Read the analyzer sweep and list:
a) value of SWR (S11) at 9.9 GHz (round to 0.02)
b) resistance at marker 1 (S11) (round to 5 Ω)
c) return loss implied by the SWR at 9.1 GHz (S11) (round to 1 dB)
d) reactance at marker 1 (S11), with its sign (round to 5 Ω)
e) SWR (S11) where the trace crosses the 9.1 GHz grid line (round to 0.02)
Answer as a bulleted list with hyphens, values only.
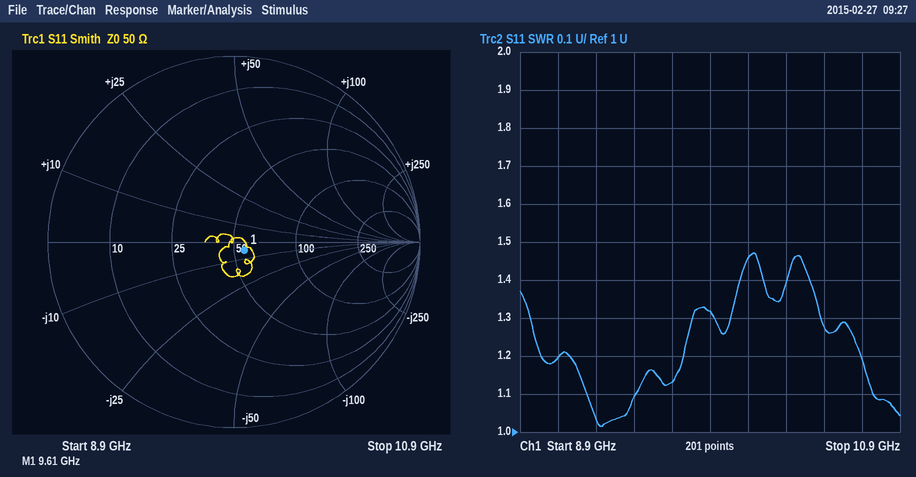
- 1.32
- 55 Ω
- 21 dB
- -5 Ω
- 1.20
